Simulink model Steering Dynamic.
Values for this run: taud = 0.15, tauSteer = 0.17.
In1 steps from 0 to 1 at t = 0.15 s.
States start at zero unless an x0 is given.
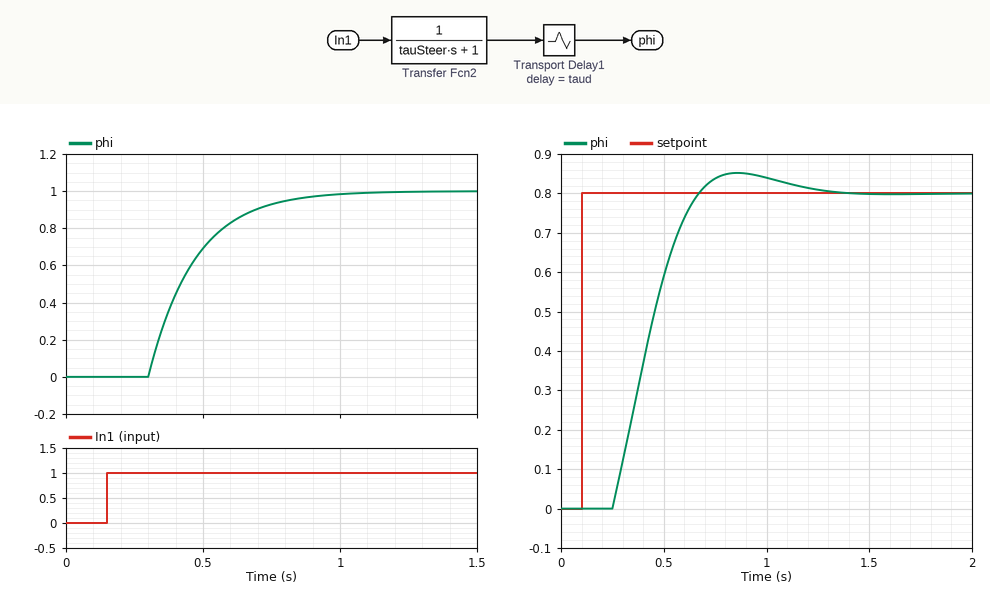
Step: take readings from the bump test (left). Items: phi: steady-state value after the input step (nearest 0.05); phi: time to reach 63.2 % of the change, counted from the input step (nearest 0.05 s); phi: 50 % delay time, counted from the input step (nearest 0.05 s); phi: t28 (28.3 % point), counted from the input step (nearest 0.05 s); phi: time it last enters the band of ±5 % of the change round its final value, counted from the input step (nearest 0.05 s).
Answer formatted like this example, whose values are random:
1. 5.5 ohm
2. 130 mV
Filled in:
1. 1.00
2. 0.30 s
3. 0.25 s
4. 0.20 s
5. 0.65 s
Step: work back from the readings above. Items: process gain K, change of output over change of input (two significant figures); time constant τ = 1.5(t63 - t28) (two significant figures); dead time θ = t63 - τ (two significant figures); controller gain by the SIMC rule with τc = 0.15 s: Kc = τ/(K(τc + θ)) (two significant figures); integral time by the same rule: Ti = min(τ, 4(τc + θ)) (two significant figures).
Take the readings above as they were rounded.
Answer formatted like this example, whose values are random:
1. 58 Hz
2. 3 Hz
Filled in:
1. 1.0
2. 0.15 s
3. 0.15 s
4. 0.50
5. 0.15 s
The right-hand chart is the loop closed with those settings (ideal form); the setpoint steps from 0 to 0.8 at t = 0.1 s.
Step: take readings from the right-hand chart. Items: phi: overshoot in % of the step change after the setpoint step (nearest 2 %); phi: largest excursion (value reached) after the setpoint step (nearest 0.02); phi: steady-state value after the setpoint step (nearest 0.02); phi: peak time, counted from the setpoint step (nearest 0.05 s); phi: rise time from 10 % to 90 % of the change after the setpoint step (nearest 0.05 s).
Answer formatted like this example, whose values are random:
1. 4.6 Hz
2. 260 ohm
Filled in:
1. 6 %
2. 0.86
3. 0.80
4. 0.75 s
5. 0.30 s
